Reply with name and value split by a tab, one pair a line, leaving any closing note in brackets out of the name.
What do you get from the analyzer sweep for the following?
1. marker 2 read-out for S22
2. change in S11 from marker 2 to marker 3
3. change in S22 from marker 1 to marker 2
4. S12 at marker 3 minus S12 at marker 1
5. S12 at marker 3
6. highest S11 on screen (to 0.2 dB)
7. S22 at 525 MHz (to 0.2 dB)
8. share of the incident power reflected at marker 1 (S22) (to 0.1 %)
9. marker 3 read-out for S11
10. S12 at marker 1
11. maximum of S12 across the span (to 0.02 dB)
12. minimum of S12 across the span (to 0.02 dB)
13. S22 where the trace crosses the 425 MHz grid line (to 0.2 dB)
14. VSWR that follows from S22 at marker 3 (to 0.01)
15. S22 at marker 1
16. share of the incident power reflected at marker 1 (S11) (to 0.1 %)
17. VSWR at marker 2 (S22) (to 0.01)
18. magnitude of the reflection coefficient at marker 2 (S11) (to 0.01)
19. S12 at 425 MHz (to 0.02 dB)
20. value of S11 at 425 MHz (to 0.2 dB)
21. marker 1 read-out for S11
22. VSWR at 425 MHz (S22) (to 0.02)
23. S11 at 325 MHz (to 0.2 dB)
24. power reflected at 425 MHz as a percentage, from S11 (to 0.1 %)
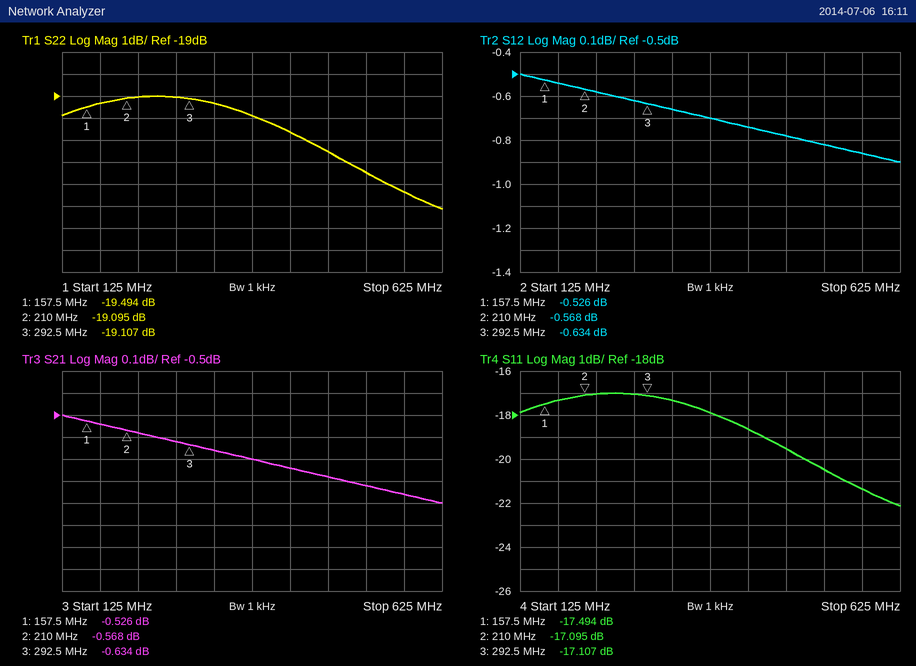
marker 2 read-out for S22	-19.095 dB
change in S11 from marker 2 to marker 3	-0.012 dB
change in S22 from marker 1 to marker 2	0.399 dB
S12 at marker 3 minus S12 at marker 1	-0.108 dB
S12 at marker 3	-0.634 dB
highest S11 on screen	-17.0 dB
S22 at 525 MHz	-22.4 dB
share of the incident power reflected at marker 1 (S22)	1.1 %
marker 3 read-out for S11	-17.107 dB
S12 at marker 1	-0.526 dB
maximum of S12 across the span	-0.50 dB
minimum of S12 across the span	-0.90 dB
S22 where the trace crosses the 425 MHz grid line	-20.6 dB
VSWR that follows from S22 at marker 3	1.25
S22 at marker 1	-19.494 dB
share of the incident power reflected at marker 1 (S11)	1.8 %
VSWR at marker 2 (S22)	1.25
magnitude of the reflection coefficient at marker 2 (S11)	0.14
S12 at 425 MHz	-0.74 dB
value of S11 at 425 MHz	-18.6 dB
marker 1 read-out for S11	-17.494 dB
VSWR at 425 MHz (S22)	1.20
S11 at 325 MHz	-17.4 dB
power reflected at 425 MHz as a percentage, from S11	1.4 %
